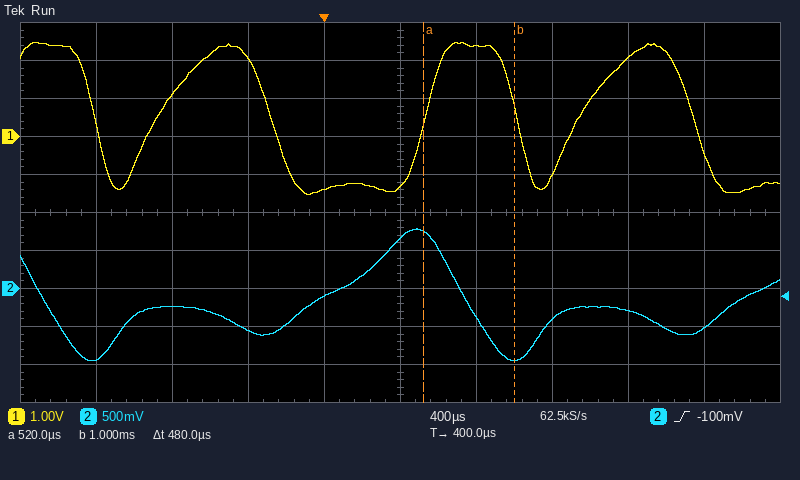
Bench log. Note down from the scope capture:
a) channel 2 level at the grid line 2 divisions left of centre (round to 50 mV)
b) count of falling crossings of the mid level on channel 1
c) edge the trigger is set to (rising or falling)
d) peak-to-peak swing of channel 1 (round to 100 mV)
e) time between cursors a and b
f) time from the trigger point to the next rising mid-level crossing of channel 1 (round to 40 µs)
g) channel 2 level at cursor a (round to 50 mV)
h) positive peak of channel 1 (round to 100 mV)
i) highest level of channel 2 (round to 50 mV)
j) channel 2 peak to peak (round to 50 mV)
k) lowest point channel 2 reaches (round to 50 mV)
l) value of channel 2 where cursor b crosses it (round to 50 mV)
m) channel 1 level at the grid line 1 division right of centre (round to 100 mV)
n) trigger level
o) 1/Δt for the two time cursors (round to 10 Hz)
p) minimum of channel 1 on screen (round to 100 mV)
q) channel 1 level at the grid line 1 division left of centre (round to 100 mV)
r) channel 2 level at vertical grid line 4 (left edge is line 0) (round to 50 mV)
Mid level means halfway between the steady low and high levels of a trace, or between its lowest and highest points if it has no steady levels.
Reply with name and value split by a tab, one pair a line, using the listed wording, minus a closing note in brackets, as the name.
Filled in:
channel 2 level at the grid line 2 divisions left of centre	-550 mV
count of falling crossings of the mid level on channel 1	4
edge the trigger is set to	rising
peak-to-peak swing of channel 1	4.0 V
time between cursors a and b	480 µs
time from the trigger point to the next rising mid-level crossing of channel 1	520 µs
channel 2 level at cursor a	750 mV
positive peak of channel 1	2.5 V
highest level of channel 2	800 mV
channel 2 peak to peak	1.75 V
lowest point channel 2 reaches	-950 mV
value of channel 2 where cursor b crosses it	-950 mV
channel 1 level at the grid line 1 division right of centre	2.4 V
trigger level	-100 mV
1/Δt for the two time cursors	2.08 kHz
minimum of channel 1 on screen	-1.5 V
channel 1 level at the grid line 1 division left of centre	-1.4 V
channel 2 level at vertical grid line 4 (left edge is line 0)	-100 mV
